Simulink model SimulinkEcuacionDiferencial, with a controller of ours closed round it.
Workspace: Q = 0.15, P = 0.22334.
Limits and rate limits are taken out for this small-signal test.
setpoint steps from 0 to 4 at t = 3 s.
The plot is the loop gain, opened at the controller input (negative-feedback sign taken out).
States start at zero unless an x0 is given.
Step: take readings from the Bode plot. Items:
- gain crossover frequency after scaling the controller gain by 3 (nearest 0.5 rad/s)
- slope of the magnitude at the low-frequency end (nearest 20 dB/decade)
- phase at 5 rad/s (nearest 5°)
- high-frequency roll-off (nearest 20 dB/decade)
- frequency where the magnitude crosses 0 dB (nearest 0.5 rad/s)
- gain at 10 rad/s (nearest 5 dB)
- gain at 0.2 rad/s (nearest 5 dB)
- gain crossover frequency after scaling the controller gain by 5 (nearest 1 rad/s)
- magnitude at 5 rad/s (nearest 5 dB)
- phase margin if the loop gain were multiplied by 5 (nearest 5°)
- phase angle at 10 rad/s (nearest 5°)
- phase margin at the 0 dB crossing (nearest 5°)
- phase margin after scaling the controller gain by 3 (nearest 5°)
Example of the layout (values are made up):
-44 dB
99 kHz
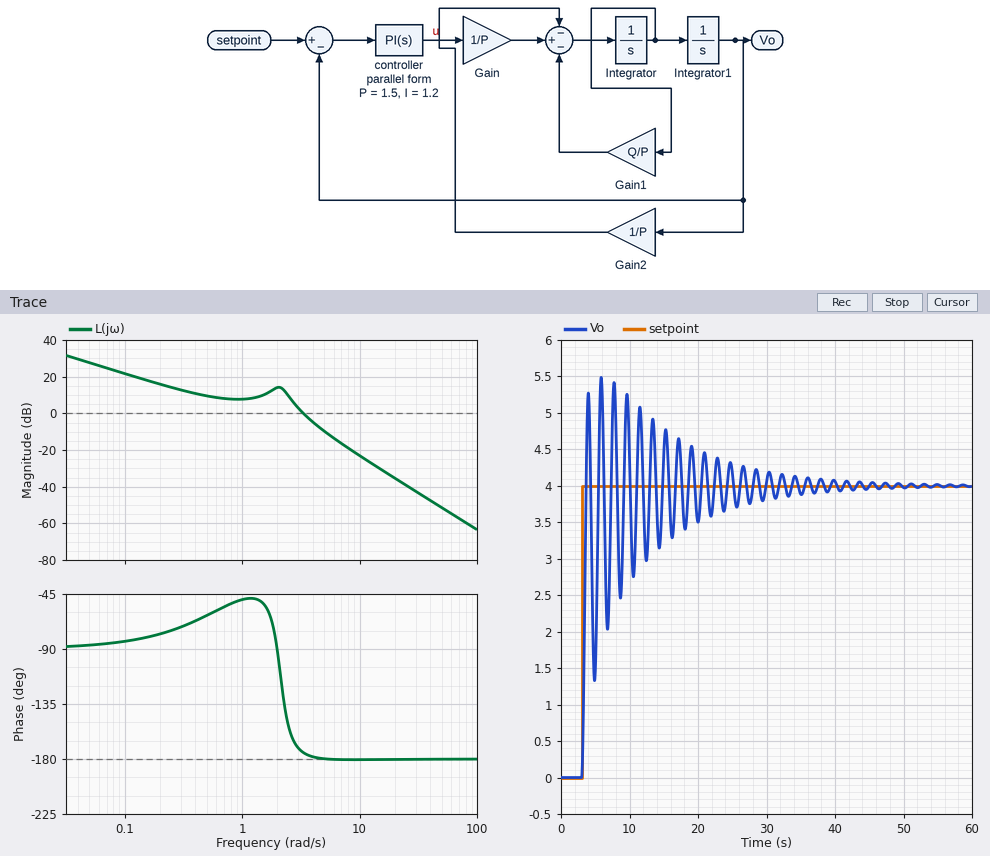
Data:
5.0 rad/s
-20 dB/decade
-180°
-40 dB/decade
3.5 rad/s
-25 dB
15 dB
6 rad/s
-10 dB
0°
-180°
5°
0°
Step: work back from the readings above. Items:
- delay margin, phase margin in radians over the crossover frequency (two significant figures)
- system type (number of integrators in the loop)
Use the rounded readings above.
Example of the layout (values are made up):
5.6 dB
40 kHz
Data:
0.025 s
1
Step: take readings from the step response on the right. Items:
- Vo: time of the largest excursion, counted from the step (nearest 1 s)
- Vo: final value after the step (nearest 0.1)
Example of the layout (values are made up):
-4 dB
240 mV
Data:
3 s
4.0
